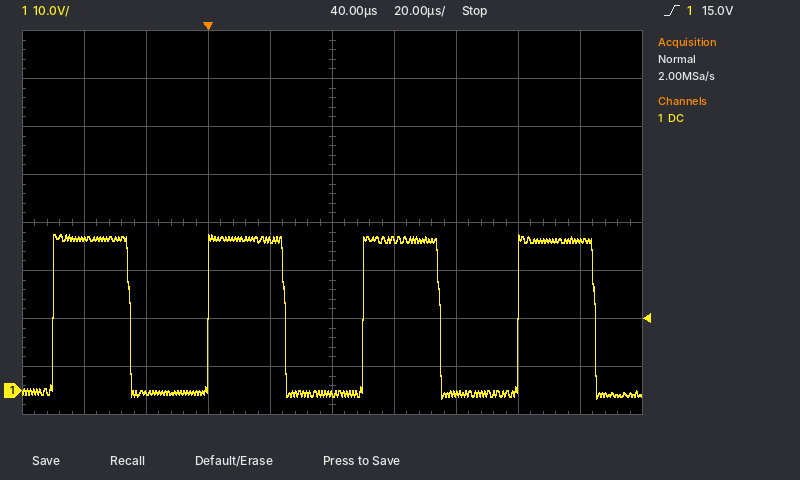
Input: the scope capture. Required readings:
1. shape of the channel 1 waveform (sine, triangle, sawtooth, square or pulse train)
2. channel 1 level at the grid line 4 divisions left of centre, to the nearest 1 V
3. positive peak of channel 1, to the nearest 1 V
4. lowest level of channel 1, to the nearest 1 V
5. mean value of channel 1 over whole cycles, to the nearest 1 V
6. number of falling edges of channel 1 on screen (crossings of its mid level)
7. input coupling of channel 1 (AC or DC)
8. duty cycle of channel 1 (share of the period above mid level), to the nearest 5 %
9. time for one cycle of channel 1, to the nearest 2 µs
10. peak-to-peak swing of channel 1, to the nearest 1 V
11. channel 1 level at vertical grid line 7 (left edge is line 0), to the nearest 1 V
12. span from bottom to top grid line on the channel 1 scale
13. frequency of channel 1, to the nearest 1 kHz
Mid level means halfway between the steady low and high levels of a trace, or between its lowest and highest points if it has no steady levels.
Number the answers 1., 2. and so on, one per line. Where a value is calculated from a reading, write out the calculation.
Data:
1. square
2. 32 V
3. 32 V
4. -2 V
5. -2 V + 0.5 × (32 V − (-2 V)) ≈ 15 V
6. 4
7. DC
8. 50 %
9. 50 µs
10. 32 V − (-2 V) = 34 V
11. -1 V
12. 80 V
13. 1 / 50 µs ≈ 20 kHz
